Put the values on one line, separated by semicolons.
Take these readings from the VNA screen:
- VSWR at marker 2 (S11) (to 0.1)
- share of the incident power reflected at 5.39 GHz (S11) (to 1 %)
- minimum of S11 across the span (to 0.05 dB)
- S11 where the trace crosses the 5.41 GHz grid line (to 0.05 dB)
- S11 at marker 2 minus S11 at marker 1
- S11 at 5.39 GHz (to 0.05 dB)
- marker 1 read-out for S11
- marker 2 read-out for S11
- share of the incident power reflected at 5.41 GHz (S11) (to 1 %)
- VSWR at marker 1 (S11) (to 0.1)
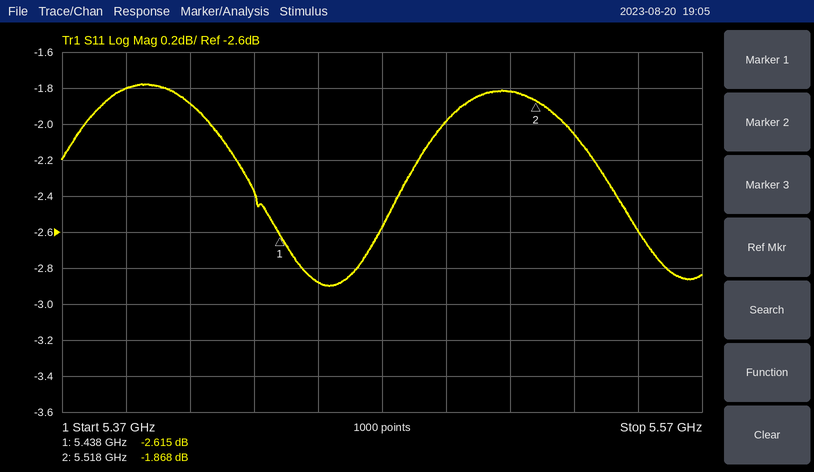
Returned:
9.3; 66 %; -2.90 dB; -1.90 dB; 0.747 dB; -1.80 dB; -2.615 dB; -1.868 dB; 65 %; 6.7
